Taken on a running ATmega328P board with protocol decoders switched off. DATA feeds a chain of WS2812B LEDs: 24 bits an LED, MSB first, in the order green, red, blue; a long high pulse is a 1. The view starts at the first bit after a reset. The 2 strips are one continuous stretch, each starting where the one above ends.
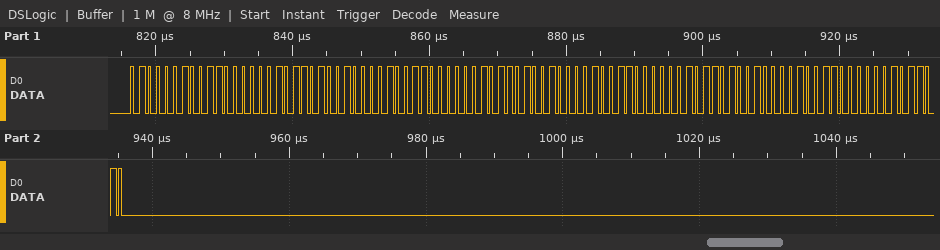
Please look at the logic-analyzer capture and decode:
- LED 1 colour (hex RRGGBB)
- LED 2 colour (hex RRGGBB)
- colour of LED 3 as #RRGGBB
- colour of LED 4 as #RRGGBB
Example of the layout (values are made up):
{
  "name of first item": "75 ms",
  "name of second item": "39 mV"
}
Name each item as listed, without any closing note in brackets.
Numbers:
{
  "LED 1 colour": "#60425A",
  "LED 2 colour": "#60425A",
  "colour of LED 3 as #RRGGBB": "#60425A",
  "colour of LED 4 as #RRGGBB": "#60425A"
}
